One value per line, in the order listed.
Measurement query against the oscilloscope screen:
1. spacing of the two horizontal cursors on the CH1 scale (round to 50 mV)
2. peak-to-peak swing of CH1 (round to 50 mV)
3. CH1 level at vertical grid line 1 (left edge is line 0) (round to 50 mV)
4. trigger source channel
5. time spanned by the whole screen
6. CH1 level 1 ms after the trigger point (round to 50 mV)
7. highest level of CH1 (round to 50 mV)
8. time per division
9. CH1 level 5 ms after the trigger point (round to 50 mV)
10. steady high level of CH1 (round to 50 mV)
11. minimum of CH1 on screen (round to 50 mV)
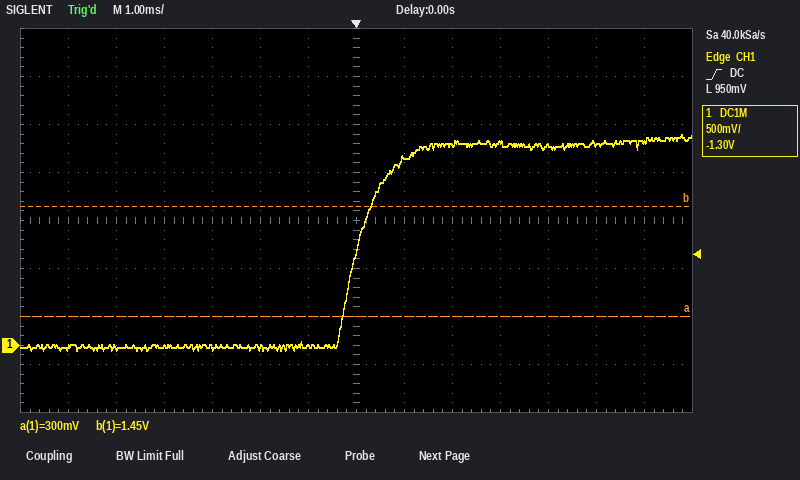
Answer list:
1.15 V
2.25 V
0 mV
CH1
14 ms
1.95 V
2.20 V
1 ms
2.10 V
2.10 V
-50 mV
